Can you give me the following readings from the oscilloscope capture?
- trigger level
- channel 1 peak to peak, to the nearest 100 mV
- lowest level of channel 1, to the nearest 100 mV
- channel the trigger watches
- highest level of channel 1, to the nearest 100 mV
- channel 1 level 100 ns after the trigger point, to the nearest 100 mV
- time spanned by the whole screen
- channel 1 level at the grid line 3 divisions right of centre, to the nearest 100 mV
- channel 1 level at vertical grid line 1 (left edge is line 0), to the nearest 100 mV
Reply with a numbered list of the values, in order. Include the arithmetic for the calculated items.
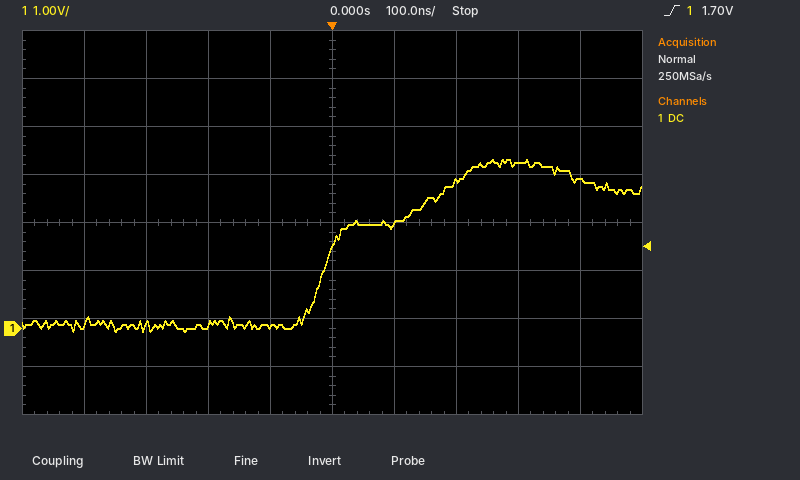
1. 1.70 V
2. 3.5 V − (-100 mV) = 3.6 V
3. -100 mV
4. channel 1
5. 3.5 V
6. 2.2 V
7. 1 µs
8. 3.4 V
9. 100 mV
